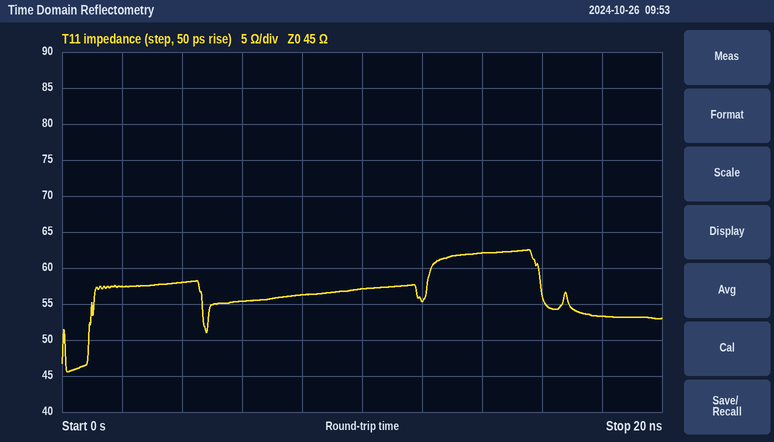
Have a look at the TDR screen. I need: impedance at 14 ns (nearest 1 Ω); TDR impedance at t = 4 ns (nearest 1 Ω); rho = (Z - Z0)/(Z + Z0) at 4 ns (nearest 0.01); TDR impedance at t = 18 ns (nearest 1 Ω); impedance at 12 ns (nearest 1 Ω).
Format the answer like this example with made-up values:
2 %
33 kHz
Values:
62 Ω
58 Ω
+0.13
53 Ω
55 Ω
